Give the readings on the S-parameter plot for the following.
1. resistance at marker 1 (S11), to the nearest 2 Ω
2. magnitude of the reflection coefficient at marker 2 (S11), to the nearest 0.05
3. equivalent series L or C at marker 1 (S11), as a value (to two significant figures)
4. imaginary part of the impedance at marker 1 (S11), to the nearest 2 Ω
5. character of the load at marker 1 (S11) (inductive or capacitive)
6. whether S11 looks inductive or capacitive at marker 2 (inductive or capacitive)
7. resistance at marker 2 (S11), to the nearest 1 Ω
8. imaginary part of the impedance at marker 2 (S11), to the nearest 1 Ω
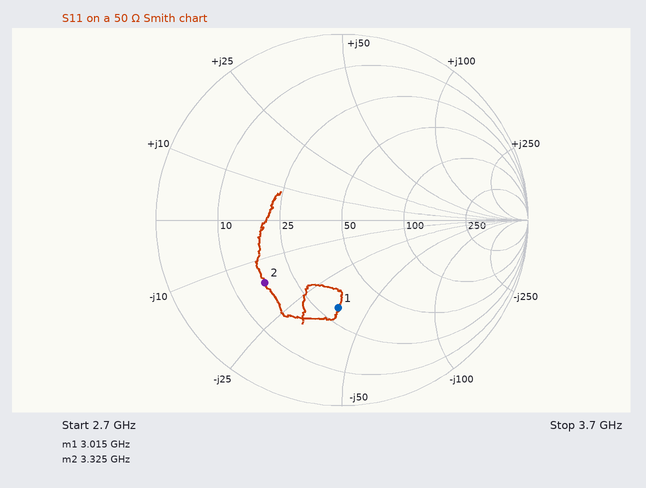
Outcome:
30 Ω
0.55
1.4 pF
-38 Ω
capacitive
capacitive
17 Ω
-16 Ω
